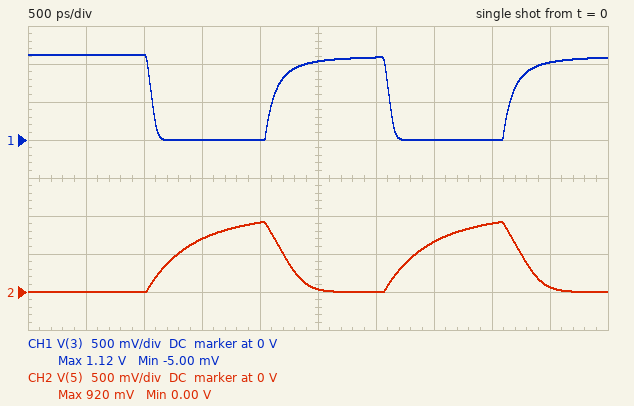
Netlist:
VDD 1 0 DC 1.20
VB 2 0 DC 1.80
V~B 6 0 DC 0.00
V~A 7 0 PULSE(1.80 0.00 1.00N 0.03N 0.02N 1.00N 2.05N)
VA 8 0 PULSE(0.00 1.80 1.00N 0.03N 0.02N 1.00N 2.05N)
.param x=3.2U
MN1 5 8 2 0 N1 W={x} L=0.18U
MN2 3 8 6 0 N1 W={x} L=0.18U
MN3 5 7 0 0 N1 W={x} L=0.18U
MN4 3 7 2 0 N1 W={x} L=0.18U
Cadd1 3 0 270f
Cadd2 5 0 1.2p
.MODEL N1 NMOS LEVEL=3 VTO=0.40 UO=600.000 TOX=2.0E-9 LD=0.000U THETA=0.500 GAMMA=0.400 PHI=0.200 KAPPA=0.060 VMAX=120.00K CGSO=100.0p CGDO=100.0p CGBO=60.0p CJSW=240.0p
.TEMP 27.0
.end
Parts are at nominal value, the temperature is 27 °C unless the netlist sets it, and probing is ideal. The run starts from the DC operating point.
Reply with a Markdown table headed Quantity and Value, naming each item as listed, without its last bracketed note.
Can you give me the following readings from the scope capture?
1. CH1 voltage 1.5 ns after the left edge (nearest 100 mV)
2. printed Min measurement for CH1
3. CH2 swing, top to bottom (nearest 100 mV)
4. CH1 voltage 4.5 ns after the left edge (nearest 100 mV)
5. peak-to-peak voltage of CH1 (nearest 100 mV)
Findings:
| Quantity | Value |
|---|---|
| CH1 voltage 1.5 ns after the left edge | 0 V |
| printed Min measurement for CH1 | -5.00 mV |
| CH2 swing, top to bottom | 900 mV |
| CH1 voltage 4.5 ns after the left edge | 1.0 V |
| peak-to-peak voltage of CH1 | 1.1 V |
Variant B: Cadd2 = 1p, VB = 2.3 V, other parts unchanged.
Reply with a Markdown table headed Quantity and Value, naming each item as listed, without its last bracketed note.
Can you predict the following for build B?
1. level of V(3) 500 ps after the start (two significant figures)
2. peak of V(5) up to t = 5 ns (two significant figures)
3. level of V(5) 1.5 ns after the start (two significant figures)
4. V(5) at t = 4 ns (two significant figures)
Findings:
| Quantity | Value |
|---|---|
| level of V(3) 500 ps after the start | 1.1 V |
| peak of V(5) up to t = 5 ns | 960 mV |
| level of V(5) 1.5 ns after the start | 760 mV |
| V(5) at t = 4 ns | 940 mV |
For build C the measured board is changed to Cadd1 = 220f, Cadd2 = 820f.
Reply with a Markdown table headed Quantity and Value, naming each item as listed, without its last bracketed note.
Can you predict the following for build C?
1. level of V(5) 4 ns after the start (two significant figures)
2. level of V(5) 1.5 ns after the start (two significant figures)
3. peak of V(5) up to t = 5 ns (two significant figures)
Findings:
| Quantity | Value |
|---|---|
| level of V(5) 4 ns after the start | 980 mV |
| level of V(5) 1.5 ns after the start | 820 mV |
| peak of V(5) up to t = 5 ns | 990 mV |
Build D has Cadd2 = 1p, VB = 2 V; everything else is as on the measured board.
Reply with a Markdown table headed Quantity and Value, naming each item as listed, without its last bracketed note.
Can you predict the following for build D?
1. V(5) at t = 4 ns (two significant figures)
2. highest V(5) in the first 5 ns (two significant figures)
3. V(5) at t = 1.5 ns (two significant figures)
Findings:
| Quantity | Value |
|---|---|
| V(5) at t = 4 ns | 940 mV |
| highest V(5) in the first 5 ns | 960 mV |
| V(5) at t = 1.5 ns | 760 mV |
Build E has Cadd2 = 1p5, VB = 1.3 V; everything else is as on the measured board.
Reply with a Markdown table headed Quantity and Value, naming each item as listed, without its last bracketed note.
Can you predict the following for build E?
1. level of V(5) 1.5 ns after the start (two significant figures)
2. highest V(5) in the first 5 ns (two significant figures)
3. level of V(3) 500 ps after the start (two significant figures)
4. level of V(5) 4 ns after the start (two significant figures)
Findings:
| Quantity | Value |
|---|---|
| level of V(5) 1.5 ns after the start | 620 mV |
| highest V(5) in the first 5 ns | 860 mV |
| level of V(3) 500 ps after the start | 1.1 V |
| level of V(5) 4 ns after the start | 840 mV |
